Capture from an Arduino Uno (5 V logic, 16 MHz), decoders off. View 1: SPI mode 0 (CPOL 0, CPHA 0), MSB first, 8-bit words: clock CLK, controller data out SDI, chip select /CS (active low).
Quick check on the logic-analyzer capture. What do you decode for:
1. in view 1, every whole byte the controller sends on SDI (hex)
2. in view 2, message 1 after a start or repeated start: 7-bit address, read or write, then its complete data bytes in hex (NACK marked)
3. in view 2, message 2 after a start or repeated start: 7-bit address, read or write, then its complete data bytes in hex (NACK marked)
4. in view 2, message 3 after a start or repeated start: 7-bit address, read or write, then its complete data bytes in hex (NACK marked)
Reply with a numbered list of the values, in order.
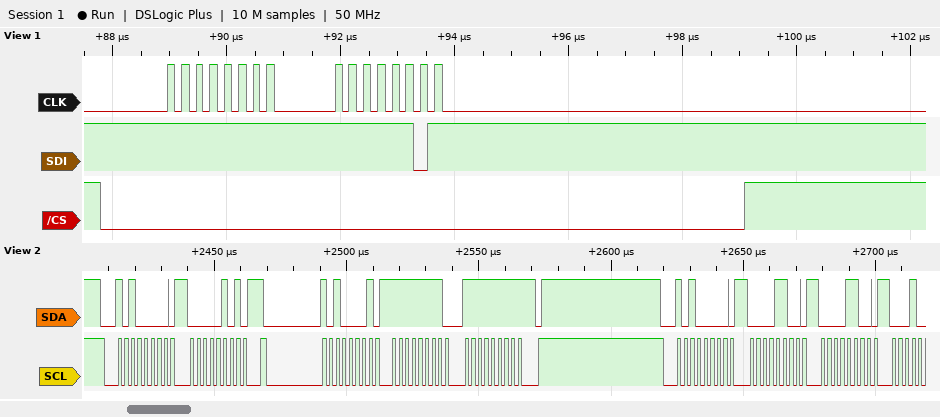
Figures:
1. FF FD
2. 0x50 write: 05
3. 0x50 read: FF FF NACK
4. 0x50 write: 0C 0C
